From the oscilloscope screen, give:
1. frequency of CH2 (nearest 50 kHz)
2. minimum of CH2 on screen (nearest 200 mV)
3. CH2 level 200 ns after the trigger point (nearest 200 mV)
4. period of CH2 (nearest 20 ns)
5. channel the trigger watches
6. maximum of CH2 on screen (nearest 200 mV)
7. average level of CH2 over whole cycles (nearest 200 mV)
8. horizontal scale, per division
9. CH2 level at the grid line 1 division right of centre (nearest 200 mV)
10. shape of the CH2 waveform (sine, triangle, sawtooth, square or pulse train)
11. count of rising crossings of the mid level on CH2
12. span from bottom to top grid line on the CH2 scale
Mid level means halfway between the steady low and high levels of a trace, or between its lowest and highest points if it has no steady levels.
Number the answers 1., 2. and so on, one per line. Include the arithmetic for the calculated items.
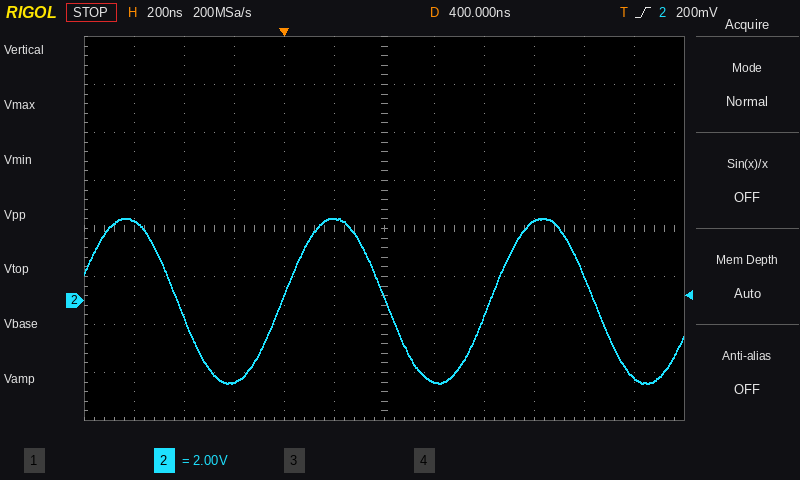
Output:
1. 1 / 840 ns ≈ 1.19 MHz, so 1.20 MHz to the nearest 50 kHz
2. -3.4 V
3. 3.4 V
4. 840 ns
5. CH2
6. 3.4 V
7. (3.4 V + (-3.4 V)) / 2 ≈ 0.0 V
8. 200 ns
9. -3.4 V
10. sine
11. 2
12. 16 V
